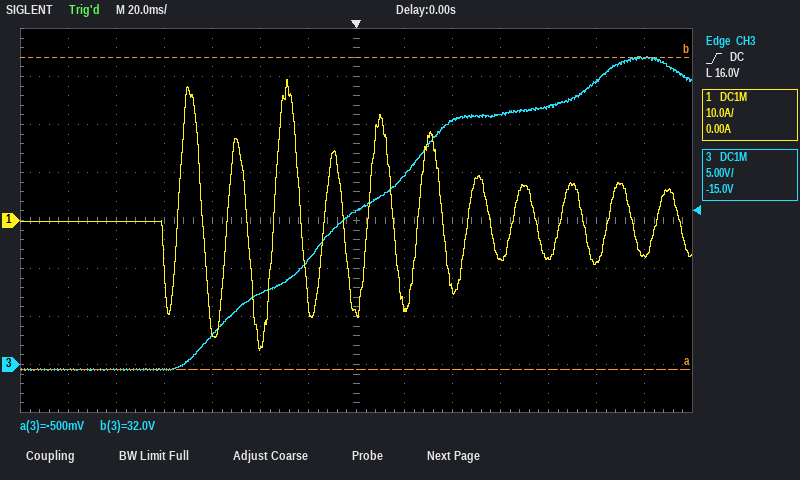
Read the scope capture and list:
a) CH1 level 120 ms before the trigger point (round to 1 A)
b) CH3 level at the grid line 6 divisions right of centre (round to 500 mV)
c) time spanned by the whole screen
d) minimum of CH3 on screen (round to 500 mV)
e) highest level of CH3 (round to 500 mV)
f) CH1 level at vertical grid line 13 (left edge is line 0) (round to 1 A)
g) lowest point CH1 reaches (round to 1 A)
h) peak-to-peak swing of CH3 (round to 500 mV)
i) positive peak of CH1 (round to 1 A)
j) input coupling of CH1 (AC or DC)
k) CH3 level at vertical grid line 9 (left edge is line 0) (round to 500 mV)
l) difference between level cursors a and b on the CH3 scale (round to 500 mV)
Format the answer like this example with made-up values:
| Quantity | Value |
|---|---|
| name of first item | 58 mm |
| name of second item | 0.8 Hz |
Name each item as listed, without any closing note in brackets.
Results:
| Quantity | Value |
|---|---|
| CH1 level 120 ms before the trigger point | 0 A |
| CH3 level at the grid line 6 divisions right of centre | 32.0 V |
| time spanned by the whole screen | 280 ms |
| minimum of CH3 on screen | -500 mV |
| highest level of CH3 | 32.0 V |
| CH1 level at vertical grid line 13 (left edge is line 0) | -7 A |
| lowest point CH1 reaches | -27 A |
| peak-to-peak swing of CH3 | 32.5 V |
| positive peak of CH1 | 29 A |
| input coupling of CH1 | DC |
| CH3 level at vertical grid line 9 (left edge is line 0) | 25.5 V |
| difference between level cursors a and b on the CH3 scale | 32.5 V |
